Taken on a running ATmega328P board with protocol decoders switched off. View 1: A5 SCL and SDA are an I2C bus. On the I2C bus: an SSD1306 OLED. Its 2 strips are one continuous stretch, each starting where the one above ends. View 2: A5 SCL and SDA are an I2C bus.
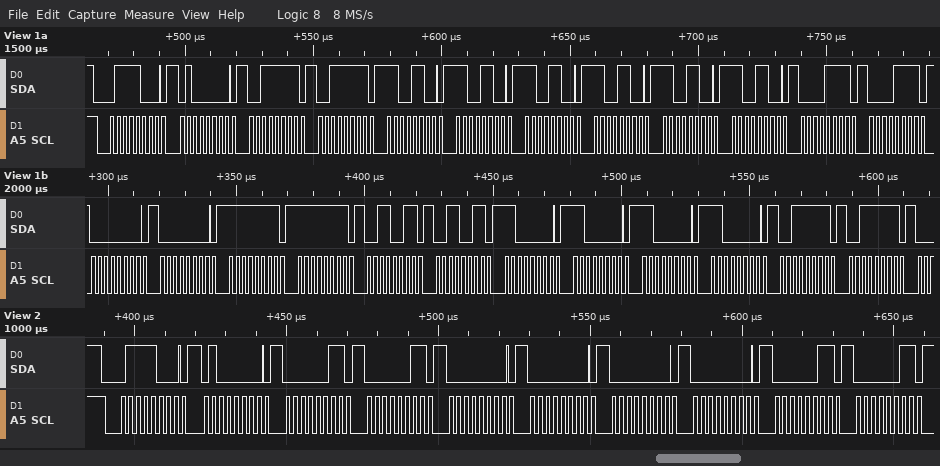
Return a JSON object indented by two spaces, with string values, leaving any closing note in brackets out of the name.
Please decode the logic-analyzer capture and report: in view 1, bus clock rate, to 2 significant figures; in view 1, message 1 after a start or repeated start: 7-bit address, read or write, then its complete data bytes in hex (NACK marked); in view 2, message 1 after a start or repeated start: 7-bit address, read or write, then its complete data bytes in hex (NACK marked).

{
  "in view 1, bus clock rate, to 2 significant figures": "400 kHz",
  "in view 1, message 1 after a start or repeated start: 7-bit address, read or write, then its complete data bytes in hex": "0x3C write: 40 3F 3F CC CC CC CC CC CC 0F 0F 00 00 FF FF 33 33 C0 C0 C0 C0 3F 3F",
  "in view 2, message 1 after a start or repeated start: 7-bit address, read or write, then its complete data bytes in hex": "0x3C write: 40 03 03 00 00 00 00 03 03"
}
